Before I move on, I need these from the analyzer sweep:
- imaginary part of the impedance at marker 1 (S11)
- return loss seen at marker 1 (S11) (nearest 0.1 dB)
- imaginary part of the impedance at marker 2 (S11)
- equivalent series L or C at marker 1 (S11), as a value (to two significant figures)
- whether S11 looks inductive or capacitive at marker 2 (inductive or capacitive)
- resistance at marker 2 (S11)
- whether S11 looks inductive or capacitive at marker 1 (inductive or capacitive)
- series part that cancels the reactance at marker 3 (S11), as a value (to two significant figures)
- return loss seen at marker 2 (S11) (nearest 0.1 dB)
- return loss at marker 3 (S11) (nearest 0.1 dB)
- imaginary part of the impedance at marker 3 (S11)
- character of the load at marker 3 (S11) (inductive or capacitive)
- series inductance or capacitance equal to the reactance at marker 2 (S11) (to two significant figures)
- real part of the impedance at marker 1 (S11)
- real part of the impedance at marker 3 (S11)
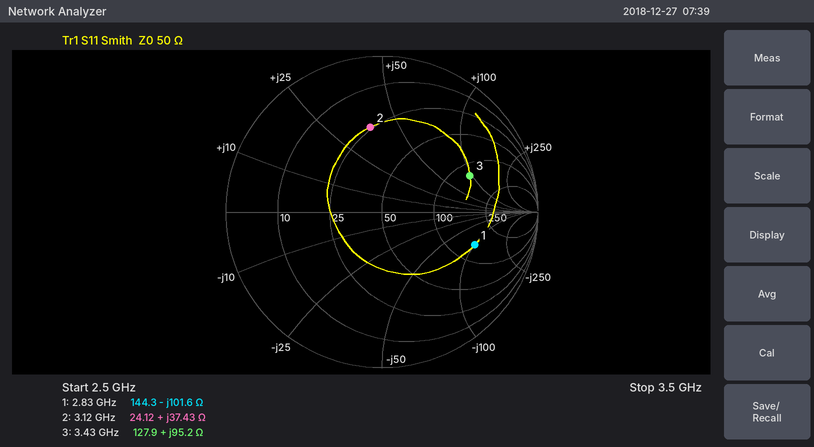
-101.6 Ω
4.0 dB
+37.43 Ω
550 fF
inductive
24.12 Ω
capacitive
490 fF
5.2 dB
4.3 dB
+95.2 Ω
inductive
1.9 nH
144.3 Ω
127.9 Ω
